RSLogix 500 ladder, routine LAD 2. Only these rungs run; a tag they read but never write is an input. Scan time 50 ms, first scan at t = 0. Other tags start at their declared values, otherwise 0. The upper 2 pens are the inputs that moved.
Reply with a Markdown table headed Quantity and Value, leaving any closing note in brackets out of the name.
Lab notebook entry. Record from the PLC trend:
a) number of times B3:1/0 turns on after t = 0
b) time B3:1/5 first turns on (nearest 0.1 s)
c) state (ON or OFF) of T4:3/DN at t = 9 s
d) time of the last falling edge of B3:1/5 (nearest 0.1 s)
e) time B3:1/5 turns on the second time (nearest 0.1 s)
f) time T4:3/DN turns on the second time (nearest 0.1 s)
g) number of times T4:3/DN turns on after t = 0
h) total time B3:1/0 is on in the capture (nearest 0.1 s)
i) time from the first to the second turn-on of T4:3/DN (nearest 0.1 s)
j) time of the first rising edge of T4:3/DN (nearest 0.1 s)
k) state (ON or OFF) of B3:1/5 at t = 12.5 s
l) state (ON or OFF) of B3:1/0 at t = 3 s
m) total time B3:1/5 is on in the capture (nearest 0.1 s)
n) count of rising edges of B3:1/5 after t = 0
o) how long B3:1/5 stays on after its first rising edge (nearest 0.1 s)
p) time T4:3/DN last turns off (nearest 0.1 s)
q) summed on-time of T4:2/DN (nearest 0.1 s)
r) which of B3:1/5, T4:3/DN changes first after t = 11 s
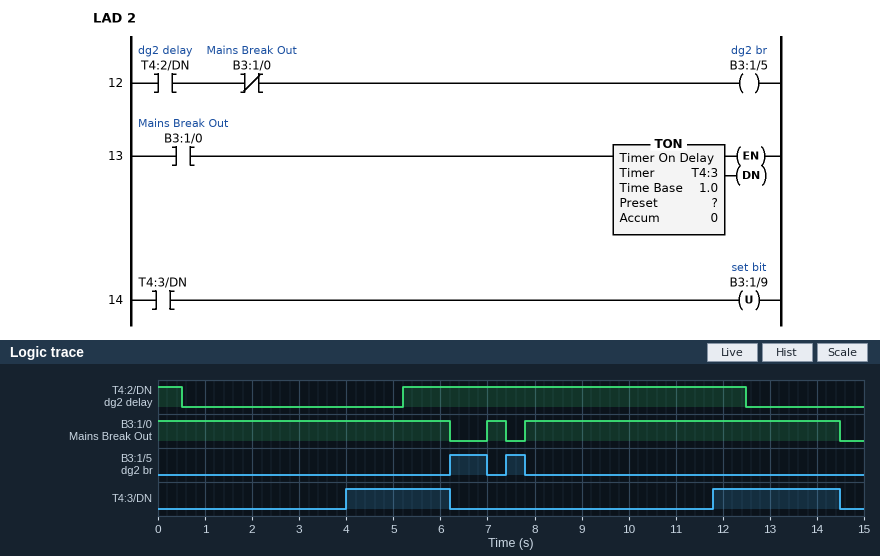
| Quantity | Value |
|---|---|
| number of times B3:1/0 turns on after t = 0 | 2 |
| time B3:1/5 first turns on | 6.2 s |
| state (ON or OFF) of T4:3/DN at t = 9 s | OFF |
| time of the last falling edge of B3:1/5 | 7.8 s |
| time B3:1/5 turns on the second time | 7.4 s |
| time T4:3/DN turns on the second time | 11.8 s |
| number of times T4:3/DN turns on after t = 0 | 2 |
| total time B3:1/0 is on in the capture | 13.3 s |
| time from the first to the second turn-on of T4:3/DN | 7.8 s |
| time of the first rising edge of T4:3/DN | 4.0 s |
| state (ON or OFF) of B3:1/5 at t = 12.5 s | OFF |
| state (ON or OFF) of B3:1/0 at t = 3 s | ON |
| total time B3:1/5 is on in the capture | 1.2 s |
| count of rising edges of B3:1/5 after t = 0 | 2 |
| how long B3:1/5 stays on after its first rising edge | 0.8 s |
| time T4:3/DN last turns off | 14.5 s |
| summed on-time of T4:2/DN | 7.8 s |
| which of B3:1/5, T4:3/DN changes first after t = 11 s | T4:3/DN |
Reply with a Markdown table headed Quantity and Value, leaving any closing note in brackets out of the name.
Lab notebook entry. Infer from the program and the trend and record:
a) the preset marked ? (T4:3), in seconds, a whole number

| Quantity | Value |
|---|---|
| the preset marked ? (T4:3), in seconds, a whole number | 4 s |
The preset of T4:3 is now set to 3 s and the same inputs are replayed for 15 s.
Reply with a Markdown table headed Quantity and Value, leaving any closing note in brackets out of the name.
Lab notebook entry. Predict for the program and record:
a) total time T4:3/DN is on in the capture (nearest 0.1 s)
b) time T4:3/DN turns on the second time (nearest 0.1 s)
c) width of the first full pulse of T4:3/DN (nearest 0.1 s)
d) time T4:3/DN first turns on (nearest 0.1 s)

| Quantity | Value |
|---|---|
| total time T4:3/DN is on in the capture | 6.9 s |
| time T4:3/DN turns on the second time | 10.8 s |
| width of the first full pulse of T4:3/DN | 3.2 s |
| time T4:3/DN first turns on | 3.0 s |
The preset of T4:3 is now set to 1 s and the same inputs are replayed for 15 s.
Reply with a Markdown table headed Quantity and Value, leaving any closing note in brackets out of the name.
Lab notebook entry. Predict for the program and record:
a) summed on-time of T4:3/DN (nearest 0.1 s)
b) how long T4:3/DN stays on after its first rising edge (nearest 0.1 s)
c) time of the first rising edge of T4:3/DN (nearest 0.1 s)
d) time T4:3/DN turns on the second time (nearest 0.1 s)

| Quantity | Value |
|---|---|
| summed on-time of T4:3/DN | 10.9 s |
| how long T4:3/DN stays on after its first rising edge | 5.2 s |
| time of the first rising edge of T4:3/DN | 1.0 s |
| time T4:3/DN turns on the second time | 8.8 s |
